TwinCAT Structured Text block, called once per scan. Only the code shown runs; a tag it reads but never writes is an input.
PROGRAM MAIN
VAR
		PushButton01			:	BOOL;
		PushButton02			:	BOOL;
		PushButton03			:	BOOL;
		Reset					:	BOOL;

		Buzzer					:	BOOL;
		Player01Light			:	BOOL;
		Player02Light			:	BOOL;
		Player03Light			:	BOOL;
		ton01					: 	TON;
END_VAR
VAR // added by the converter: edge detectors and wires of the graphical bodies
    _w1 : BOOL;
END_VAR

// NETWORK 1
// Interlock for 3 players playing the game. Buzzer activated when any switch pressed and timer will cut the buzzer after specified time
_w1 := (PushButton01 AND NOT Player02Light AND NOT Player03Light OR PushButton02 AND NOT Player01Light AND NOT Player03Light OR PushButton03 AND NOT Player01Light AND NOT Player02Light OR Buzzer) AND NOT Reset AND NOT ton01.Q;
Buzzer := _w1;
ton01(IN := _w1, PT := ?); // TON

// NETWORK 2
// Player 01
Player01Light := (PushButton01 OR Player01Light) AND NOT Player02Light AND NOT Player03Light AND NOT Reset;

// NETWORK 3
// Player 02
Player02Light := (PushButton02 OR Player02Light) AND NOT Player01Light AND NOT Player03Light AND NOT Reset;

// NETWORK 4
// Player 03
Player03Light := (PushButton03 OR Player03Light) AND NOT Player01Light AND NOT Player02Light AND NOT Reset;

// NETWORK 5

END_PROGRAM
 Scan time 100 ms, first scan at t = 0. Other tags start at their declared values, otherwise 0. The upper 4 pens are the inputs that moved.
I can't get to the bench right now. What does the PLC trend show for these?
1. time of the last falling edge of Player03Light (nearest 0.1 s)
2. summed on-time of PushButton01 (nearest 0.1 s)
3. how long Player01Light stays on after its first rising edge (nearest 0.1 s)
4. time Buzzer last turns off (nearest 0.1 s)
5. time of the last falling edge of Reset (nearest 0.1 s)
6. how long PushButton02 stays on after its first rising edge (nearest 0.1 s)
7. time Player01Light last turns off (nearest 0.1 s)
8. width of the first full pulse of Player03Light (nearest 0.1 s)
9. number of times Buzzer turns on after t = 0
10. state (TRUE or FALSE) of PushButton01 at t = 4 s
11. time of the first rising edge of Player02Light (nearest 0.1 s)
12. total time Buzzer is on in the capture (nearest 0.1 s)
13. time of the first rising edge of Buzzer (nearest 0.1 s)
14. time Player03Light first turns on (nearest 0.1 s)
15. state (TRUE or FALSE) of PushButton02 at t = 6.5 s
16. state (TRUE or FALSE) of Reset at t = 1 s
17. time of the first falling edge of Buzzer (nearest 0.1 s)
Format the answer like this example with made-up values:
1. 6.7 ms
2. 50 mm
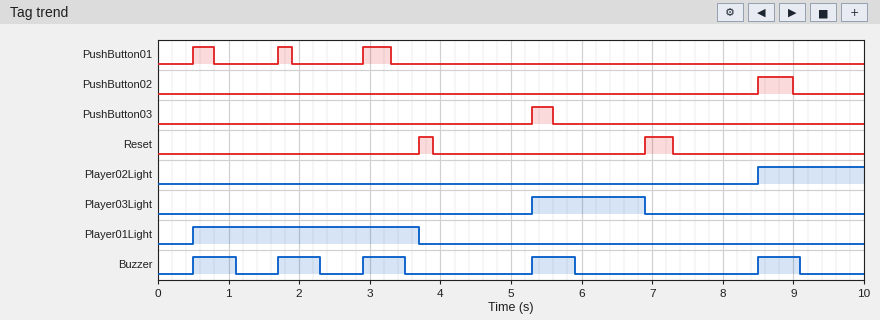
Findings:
1. 6.9 s
2. 0.9 s
3. 3.2 s
4. 9.1 s
5. 7.3 s
6. 0.5 s
7. 3.7 s
8. 1.6 s
9. 5
10. FALSE
11. 8.5 s
12. 3.0 s
13. 0.5 s
14. 5.3 s
15. FALSE
16. FALSE
17. 1.1 s
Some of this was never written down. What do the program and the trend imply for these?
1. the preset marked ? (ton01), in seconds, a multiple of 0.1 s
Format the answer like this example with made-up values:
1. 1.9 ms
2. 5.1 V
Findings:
1. 0.5 s
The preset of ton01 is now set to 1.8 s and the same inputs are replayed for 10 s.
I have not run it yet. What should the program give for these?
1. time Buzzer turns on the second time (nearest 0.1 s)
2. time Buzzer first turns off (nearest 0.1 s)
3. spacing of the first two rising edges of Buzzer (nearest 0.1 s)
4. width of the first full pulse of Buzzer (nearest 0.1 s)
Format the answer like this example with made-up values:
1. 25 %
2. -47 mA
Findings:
1. 2.9 s
2. 2.4 s
3. 2.4 s
4. 1.9 s
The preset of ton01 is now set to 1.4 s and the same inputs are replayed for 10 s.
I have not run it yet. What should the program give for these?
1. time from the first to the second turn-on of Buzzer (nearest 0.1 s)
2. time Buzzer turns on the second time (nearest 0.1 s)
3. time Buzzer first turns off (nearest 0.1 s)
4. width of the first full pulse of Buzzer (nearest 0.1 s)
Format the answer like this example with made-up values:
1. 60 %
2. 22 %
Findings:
1. 2.4 s
2. 2.9 s
3. 2.0 s
4. 1.5 s
